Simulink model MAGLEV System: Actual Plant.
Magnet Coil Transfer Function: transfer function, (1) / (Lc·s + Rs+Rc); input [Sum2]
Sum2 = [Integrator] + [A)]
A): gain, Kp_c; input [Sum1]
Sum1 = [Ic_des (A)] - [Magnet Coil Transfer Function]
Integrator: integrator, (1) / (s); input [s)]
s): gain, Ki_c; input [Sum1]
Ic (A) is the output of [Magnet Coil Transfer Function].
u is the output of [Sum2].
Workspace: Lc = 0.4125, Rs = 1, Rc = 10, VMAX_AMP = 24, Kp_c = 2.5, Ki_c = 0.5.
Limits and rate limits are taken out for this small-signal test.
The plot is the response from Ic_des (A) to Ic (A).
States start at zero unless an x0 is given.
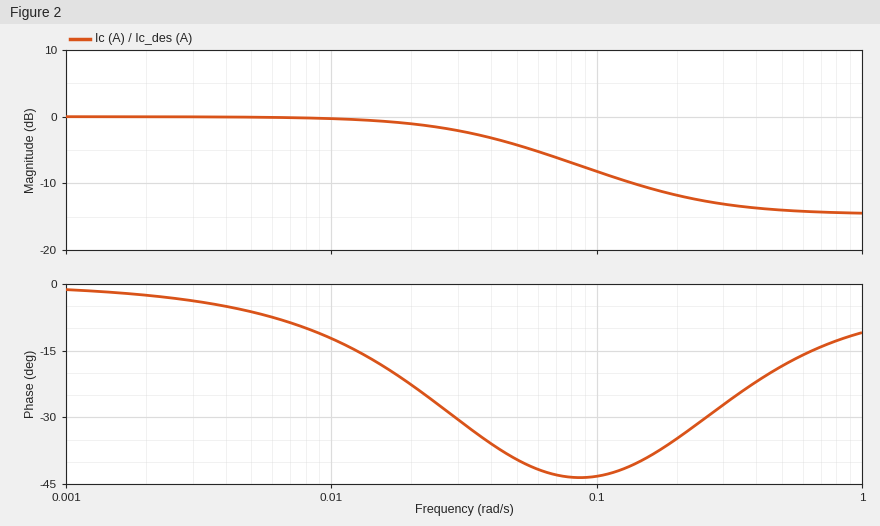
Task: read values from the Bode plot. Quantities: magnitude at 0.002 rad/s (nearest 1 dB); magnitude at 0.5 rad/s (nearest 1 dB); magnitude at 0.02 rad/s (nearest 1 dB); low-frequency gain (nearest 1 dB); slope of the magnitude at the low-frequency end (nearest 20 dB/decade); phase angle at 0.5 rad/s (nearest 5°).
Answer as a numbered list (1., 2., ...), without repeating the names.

1. 0 dB
2. -14 dB
3. -1 dB
4. 0 dB
5. 0 dB/decade
6. -20°
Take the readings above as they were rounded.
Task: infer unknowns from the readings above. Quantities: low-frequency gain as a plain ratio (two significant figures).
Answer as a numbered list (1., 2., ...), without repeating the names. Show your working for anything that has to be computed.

1. 10^(0 / 20) = 1.0
